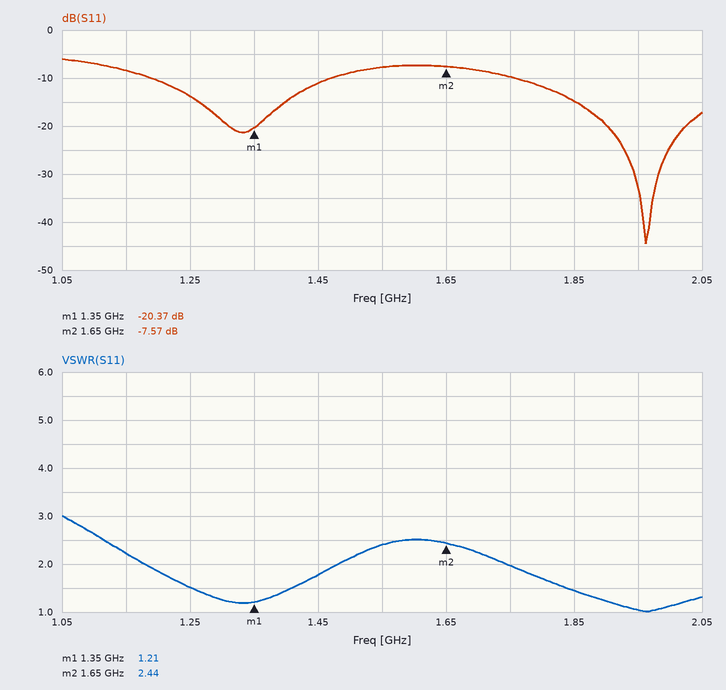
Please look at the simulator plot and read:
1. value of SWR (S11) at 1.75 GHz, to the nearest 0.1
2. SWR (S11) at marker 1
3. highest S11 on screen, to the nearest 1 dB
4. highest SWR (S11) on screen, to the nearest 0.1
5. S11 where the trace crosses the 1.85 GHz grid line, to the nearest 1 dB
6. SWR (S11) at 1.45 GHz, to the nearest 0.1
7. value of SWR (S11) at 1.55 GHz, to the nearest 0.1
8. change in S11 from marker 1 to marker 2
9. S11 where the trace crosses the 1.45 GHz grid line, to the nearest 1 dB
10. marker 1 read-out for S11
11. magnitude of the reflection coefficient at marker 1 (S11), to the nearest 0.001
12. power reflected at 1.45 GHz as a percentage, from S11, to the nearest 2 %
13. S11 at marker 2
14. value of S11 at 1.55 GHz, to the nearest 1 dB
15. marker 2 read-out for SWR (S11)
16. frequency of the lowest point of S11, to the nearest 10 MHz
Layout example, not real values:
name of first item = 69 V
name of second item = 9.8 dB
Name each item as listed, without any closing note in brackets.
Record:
value of SWR (S11) at 1.75 GHz, to the nearest 0.1 = 2.0
SWR (S11) at marker 1 = 1.21
highest S11 on screen, to the nearest 1 dB = -6 dB
highest SWR (S11) on screen, to the nearest 0.1 = 3.0
S11 where the trace crosses the 1.85 GHz grid line, to the nearest 1 dB = -15 dB
SWR (S11) at 1.45 GHz, to the nearest 0.1 = 1.8
value of SWR (S11) at 1.55 GHz, to the nearest 0.1 = 2.4
change in S11 from marker 1 to marker 2 = 12.80 dB
S11 where the trace crosses the 1.45 GHz grid line, to the nearest 1 dB = -11 dB
marker 1 read-out for S11 = -20.37 dB
magnitude of the reflection coefficient at marker 1 (S11), to the nearest 0.001 = 0.096
power reflected at 1.45 GHz as a percentage, from S11, to the nearest 2 % = 8 %
S11 at marker 2 = -7.57 dB
value of S11 at 1.55 GHz, to the nearest 1 dB = -8 dB
marker 2 read-out for SWR = 2.44
frequency of the lowest point of S11, to the nearest 10 MHz = 1.96 GHz
